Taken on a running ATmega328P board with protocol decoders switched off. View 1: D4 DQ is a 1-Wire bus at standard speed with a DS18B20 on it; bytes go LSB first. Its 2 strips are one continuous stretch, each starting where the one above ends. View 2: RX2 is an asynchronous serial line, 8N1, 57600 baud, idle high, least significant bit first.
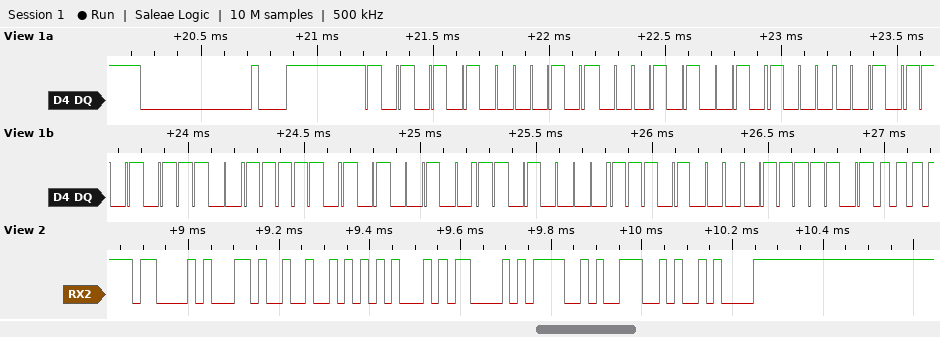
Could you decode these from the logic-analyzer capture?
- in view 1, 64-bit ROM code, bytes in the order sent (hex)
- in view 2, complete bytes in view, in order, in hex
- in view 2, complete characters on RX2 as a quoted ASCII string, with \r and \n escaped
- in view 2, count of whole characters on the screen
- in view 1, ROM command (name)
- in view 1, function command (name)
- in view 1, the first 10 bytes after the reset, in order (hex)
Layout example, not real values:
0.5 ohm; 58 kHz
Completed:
28 4A 41 EB 7C 25 0B 17; 43 2C 52 45 43 4F 4E 0A; "C,RECON\n"; 8; Match ROM; Read Scratchpad; 55 28 4A 41 EB 7C 25 0B 17 BE
